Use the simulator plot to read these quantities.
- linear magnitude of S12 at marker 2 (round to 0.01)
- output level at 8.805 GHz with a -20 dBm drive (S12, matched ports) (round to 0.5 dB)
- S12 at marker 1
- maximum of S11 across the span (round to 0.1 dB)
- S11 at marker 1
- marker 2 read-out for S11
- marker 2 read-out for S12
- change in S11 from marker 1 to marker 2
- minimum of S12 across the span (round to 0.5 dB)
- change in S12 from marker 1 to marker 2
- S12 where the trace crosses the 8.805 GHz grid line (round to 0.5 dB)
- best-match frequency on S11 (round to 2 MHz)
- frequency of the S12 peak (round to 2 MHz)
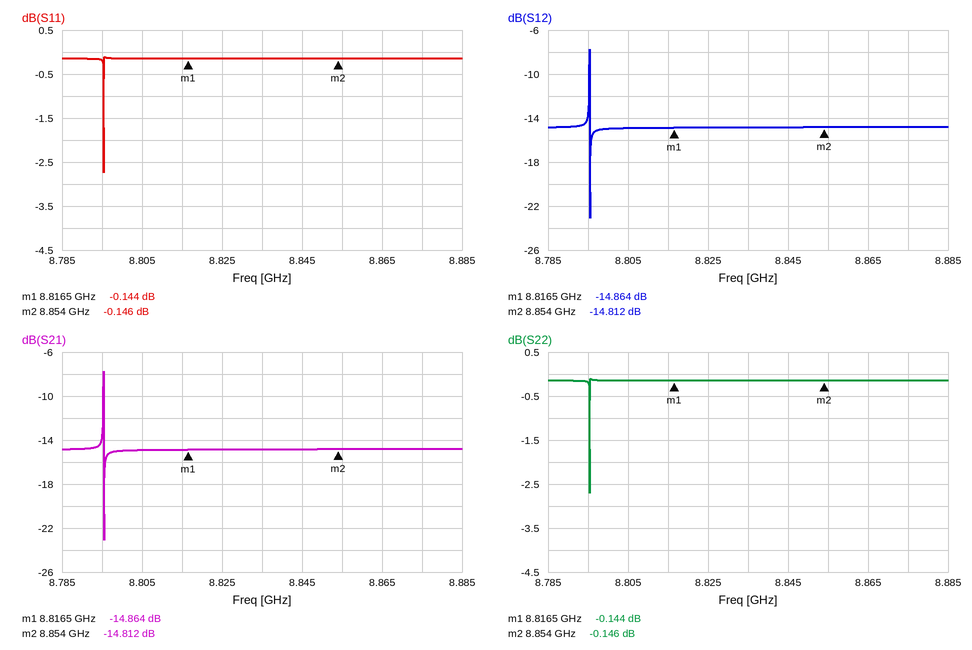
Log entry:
0.18
-35.0 dBm
-14.864 dB
-0.1 dB
-0.144 dB
-0.146 dB
-14.812 dB
-0.002 dB
-23.0 dB
0.052 dB
-15.0 dB
8.796 GHz
8.796 GHz
